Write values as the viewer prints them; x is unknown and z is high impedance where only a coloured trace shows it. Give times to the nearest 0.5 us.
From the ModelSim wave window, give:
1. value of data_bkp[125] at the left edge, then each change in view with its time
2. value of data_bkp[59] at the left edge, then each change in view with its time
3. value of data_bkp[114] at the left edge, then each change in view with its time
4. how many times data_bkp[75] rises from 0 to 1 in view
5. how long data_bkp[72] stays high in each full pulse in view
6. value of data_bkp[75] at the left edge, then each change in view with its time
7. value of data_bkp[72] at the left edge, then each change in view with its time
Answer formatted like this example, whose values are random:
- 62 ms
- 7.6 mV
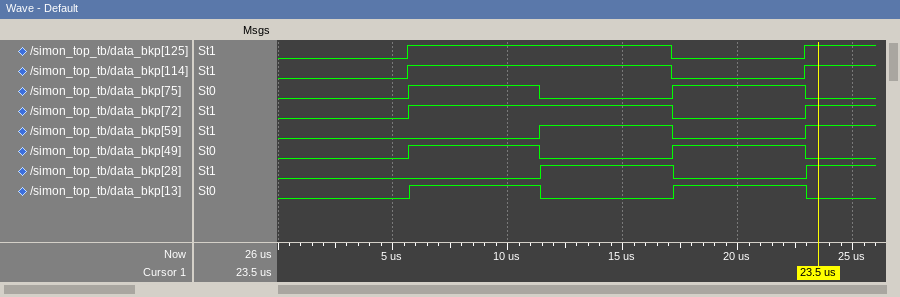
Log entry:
- 0, 1 at 5.5 us, 0 at 17 us, 1 at 23 us
- 0, 1 at 11.5 us, 0 at 17 us, 1 at 23 us
- 0, 1 at 5.5 us, 0 at 17 us, 1 at 23 us
- 2
- 11.5 us
- 0, 1 at 5.5 us, 0 at 11.5 us, 1 at 17 us, 0 at 23 us
- 0, 1 at 5.5 us, 0 at 17 us, 1 at 23 us
